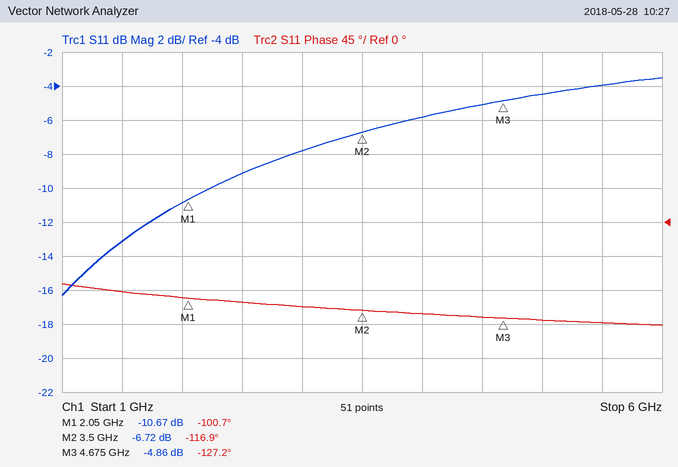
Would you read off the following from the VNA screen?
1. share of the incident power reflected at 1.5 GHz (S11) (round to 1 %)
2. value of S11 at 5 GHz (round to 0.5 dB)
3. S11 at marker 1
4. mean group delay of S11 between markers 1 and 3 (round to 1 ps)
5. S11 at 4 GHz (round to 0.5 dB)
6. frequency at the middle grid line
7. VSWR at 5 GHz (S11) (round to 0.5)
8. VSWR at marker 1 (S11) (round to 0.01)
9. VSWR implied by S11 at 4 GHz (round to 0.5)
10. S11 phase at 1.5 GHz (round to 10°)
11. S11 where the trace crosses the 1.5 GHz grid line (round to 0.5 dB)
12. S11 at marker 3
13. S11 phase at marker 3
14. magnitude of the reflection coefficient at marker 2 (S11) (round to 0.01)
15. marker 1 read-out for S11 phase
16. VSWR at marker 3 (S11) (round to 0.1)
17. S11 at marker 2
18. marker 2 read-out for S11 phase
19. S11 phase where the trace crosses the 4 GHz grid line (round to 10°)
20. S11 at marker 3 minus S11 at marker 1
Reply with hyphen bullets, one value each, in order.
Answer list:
- 5 %
- -4.5 dB
- -10.67 dB
- 28 ps
- -6.0 dB
- 3.5 GHz
- 4.0
- 1.83
- 3.0
- -90°
- -13.0 dB
- -4.86 dB
- -127.2°
- 0.46
- -100.7°
- 3.7
- -6.72 dB
- -116.9°
- -120°
- 5.81 dB
